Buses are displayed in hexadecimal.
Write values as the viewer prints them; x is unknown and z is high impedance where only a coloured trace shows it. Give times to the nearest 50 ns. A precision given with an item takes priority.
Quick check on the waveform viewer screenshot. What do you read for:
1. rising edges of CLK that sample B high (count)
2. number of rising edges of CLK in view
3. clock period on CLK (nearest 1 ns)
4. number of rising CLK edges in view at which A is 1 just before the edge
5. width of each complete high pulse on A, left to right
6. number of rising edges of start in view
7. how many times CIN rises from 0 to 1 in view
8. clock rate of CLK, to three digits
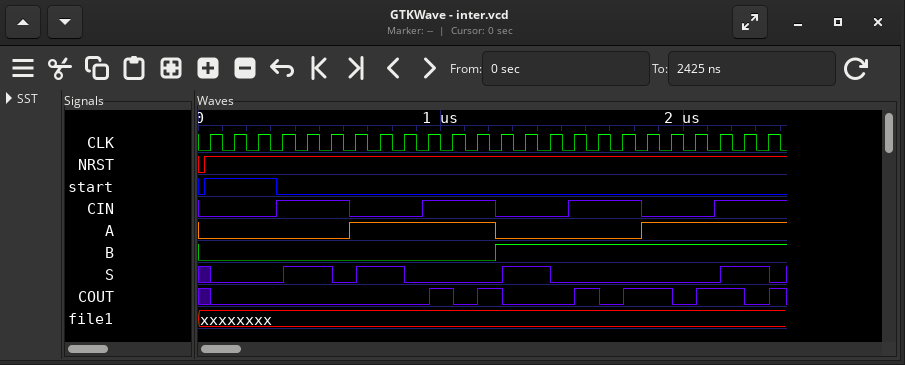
12
24
100 ns
12
600 ns
1
4
10.0 MHz
